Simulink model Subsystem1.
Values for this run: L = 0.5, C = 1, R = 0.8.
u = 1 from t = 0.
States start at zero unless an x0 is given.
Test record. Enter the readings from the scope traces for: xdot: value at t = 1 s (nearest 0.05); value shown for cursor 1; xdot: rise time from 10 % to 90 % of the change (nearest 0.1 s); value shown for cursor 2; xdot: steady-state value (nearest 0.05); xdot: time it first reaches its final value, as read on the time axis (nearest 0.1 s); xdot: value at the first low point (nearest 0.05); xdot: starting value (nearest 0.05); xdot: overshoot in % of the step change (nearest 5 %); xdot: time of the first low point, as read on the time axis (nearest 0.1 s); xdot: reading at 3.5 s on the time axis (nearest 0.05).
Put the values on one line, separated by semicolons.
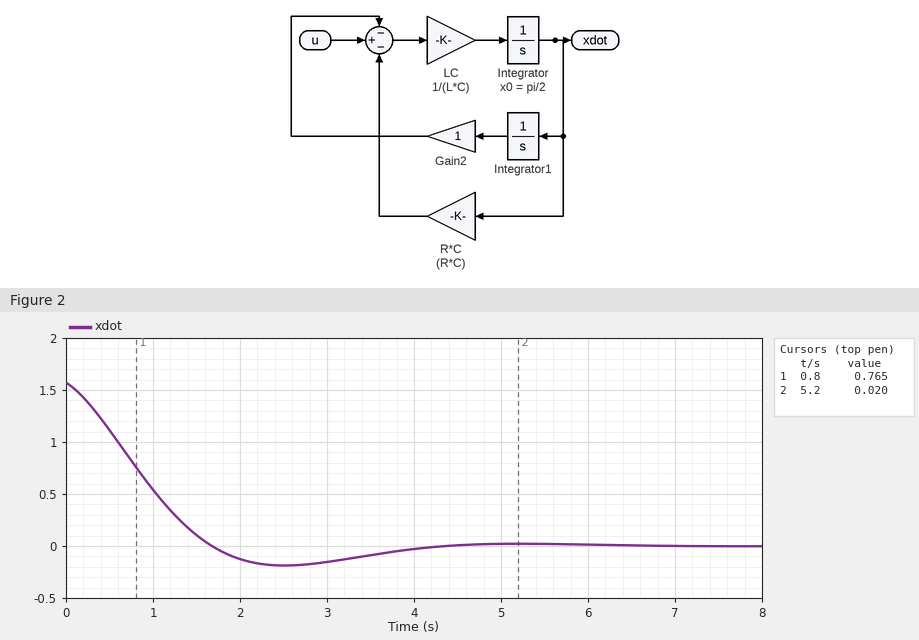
0.55; 0.765; 1.2 s; 0.020; 0.00; 1.7 s; -0.20; 1.55; 10 %; 2.5 s; -0.10
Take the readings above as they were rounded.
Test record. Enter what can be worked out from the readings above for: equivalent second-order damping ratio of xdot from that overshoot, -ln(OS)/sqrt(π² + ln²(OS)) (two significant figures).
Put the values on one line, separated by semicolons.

0.59
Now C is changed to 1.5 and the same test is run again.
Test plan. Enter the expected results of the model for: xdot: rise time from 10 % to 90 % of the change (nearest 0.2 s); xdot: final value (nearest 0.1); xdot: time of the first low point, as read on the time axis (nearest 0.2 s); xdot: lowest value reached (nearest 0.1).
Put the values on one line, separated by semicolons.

1.4 s; 0.0; 3.0 s; -0.1
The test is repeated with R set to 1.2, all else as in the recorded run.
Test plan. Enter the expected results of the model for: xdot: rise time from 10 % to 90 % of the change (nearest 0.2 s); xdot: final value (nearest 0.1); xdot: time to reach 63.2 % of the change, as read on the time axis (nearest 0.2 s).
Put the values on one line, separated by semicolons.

1.4 s; 0.0; 0.8 s
